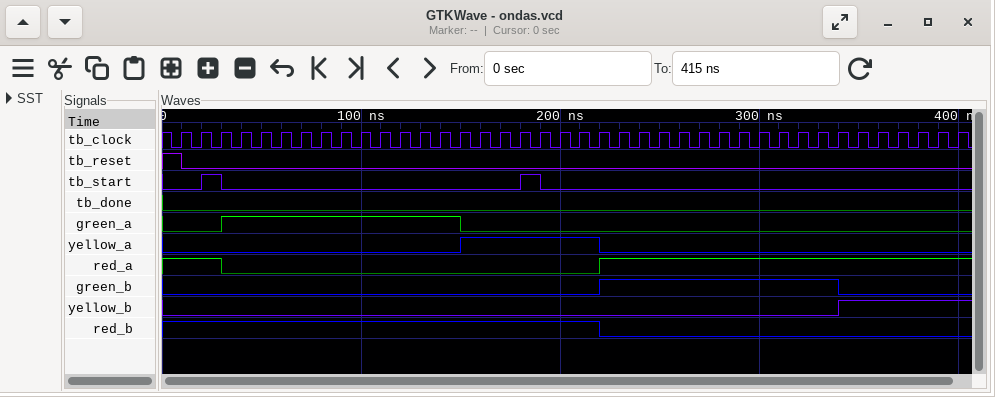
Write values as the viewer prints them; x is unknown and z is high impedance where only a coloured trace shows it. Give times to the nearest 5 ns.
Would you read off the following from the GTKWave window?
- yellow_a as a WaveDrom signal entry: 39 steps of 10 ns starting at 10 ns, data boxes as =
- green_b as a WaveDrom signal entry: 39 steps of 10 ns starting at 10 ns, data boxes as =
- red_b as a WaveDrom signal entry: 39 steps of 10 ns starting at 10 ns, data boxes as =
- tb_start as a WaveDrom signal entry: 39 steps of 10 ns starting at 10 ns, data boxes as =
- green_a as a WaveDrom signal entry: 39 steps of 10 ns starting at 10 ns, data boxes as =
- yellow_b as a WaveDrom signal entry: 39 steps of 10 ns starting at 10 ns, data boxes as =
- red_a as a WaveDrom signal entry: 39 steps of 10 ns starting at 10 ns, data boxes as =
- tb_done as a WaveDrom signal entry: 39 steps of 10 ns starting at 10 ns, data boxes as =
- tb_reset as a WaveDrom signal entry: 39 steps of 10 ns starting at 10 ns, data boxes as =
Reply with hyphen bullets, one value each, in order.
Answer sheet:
- {name: 'yellow_a', wave: '0.............1......0.................'}
- {name: 'green_b', wave: '0....................1...........0.....'}
- {name: 'red_b', wave: '1....................0.................'}
- {name: 'tb_start', wave: '010..............10....................'}
- {name: 'green_a', wave: '0.1...........0........................'}
- {name: 'yellow_b', wave: '0................................1.....'}
- {name: 'red_a', wave: '1.0..................1.................'}
- {name: 'tb_done', wave: '0......................................'}
- {name: 'tb_reset', wave: '0......................................'}
